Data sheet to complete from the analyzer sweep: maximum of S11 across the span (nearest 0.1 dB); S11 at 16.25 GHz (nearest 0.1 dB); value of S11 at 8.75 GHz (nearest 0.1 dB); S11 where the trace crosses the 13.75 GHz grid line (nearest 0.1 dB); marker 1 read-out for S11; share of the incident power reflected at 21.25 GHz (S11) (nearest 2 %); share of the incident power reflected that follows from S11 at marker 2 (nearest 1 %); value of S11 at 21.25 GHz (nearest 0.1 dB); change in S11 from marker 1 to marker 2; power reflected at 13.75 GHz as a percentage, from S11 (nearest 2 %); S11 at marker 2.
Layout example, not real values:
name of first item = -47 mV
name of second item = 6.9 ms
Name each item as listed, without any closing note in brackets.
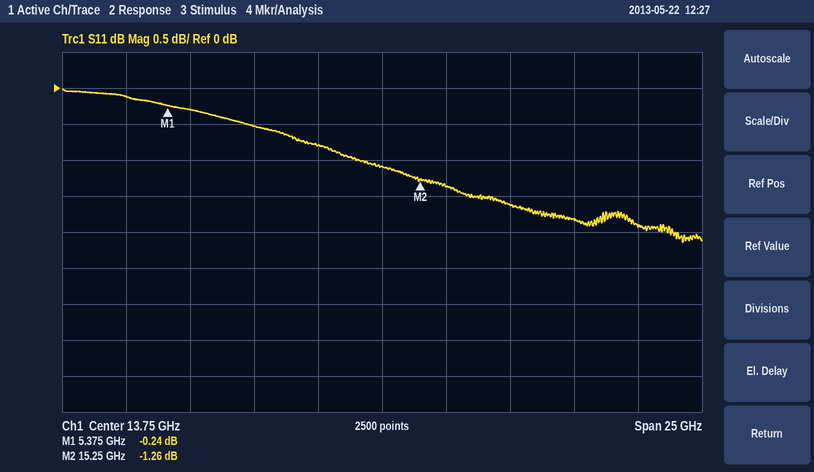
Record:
maximum of S11 across the span = 0.0 dB
S11 at 16.25 GHz = -1.4 dB
value of S11 at 8.75 GHz = -0.5 dB
S11 where the trace crosses the 13.75 GHz grid line = -1.1 dB
marker 1 read-out for S11 = -0.24 dB
share of the incident power reflected at 21.25 GHz (S11) = 66 %
share of the incident power reflected that follows from S11 at marker 2 = 75 %
value of S11 at 21.25 GHz = -1.8 dB
change in S11 from marker 1 to marker 2 = -1.02 dB
power reflected at 13.75 GHz as a percentage, from S11 = 78 %
S11 at marker 2 = -1.26 dB
